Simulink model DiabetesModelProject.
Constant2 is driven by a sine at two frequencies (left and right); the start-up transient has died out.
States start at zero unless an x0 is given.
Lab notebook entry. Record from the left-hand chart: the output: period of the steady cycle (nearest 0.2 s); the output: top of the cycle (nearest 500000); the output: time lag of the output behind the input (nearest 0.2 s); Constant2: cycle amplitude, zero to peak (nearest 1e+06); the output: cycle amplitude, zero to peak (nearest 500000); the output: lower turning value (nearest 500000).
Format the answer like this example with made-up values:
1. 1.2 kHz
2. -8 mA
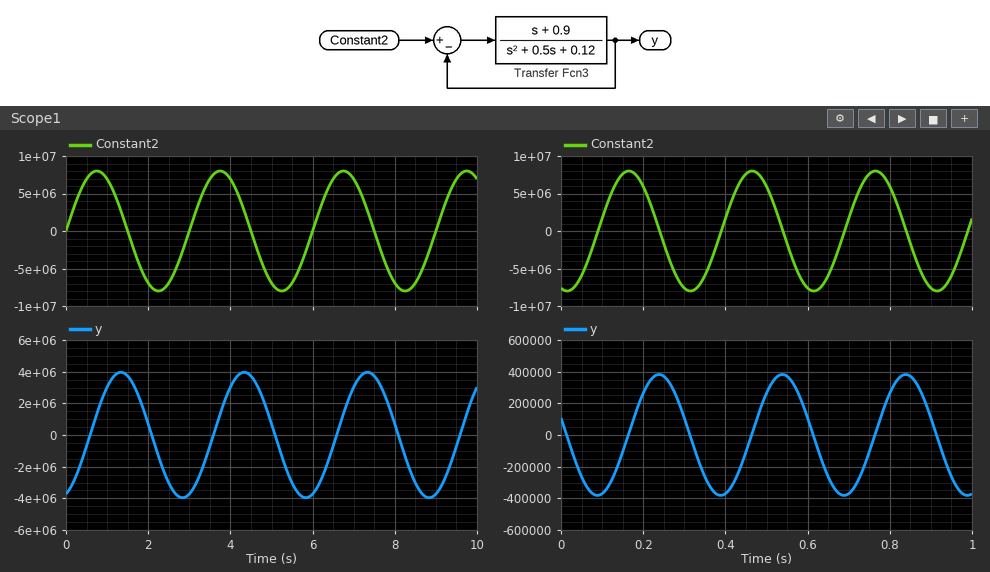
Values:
1. 3.0 s
2. 4000000
3. 0.6 s
4. 8000000
5. 4000000
6. -4000000
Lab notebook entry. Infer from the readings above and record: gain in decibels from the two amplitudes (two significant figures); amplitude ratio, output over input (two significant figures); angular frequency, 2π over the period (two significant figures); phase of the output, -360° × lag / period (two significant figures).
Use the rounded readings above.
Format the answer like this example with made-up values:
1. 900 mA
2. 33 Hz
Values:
1. -6.0 dB
2. 0.50
3. 2.1 rad/s
4. -72°
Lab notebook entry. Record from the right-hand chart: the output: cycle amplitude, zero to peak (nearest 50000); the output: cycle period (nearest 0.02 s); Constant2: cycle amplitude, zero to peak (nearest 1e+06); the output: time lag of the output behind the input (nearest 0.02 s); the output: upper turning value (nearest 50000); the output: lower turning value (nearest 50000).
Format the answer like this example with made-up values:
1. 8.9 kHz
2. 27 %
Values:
1. 400000
2. 0.30 s
3. 8000000
4. 0.08 s
5. 400000
6. -400000
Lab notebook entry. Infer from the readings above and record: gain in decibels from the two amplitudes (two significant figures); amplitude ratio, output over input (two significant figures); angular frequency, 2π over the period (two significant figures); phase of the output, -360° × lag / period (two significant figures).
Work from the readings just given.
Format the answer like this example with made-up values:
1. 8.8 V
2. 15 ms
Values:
1. -26 dB
2. 0.050
3. 21 rad/s
4. -96°
